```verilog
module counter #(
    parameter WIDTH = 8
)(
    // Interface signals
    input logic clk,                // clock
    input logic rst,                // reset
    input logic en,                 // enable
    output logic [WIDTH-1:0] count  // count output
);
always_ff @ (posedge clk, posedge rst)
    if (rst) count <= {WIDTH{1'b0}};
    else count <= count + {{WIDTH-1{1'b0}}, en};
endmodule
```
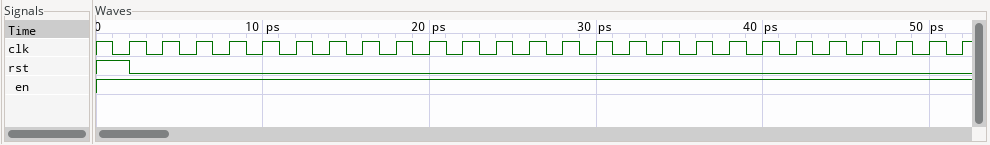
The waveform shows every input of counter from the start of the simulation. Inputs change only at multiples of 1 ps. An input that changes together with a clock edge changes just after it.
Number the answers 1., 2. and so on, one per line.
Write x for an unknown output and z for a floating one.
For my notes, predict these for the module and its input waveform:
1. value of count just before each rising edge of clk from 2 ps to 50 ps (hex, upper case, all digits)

1. 00, 00, 01, 02, 03, 04, 05, 06, 07, 08, 09, 0A, 0B, 0C, 0D, 0E, 0F, 10, 11, 12, 13, 14, 15, 16, 17
